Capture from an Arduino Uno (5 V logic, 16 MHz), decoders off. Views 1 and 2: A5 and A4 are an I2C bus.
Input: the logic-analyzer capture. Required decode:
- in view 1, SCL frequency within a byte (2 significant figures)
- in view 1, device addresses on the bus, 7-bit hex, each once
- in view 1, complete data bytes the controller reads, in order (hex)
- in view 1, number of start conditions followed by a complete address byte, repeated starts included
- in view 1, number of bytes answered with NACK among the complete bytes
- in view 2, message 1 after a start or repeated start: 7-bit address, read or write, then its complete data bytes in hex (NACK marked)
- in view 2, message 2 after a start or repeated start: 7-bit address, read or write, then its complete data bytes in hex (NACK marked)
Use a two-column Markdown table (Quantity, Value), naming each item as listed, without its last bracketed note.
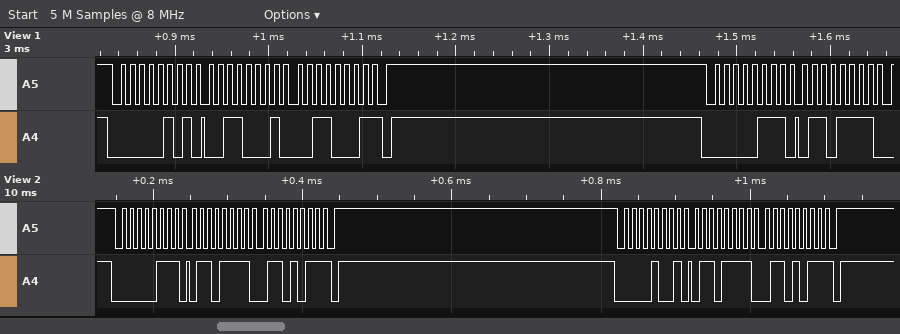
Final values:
| Quantity | Value |
|---|---|
| in view 1, SCL frequency within a byte | 100 kHz |
| in view 1, device addresses on the bus, 7-bit hex, each once | 0x02 0x03 |
| in view 1, complete data bytes the controller reads, in order | 31 31 6F |
| in view 1, number of start conditions followed by a complete address byte, repeated starts included | 2 |
| in view 1, number of bytes answered with NACK among the complete bytes | 1 |
| in view 2, message 1 after a start or repeated start: 7-bit address, read or write, then its complete data bytes in hex | 0x03 read: 6F 6B NACK |
| in view 2, message 2 after a start or repeated start: 7-bit address, read or write, then its complete data bytes in hex | 0x04 read: 6F 6B NACK |
